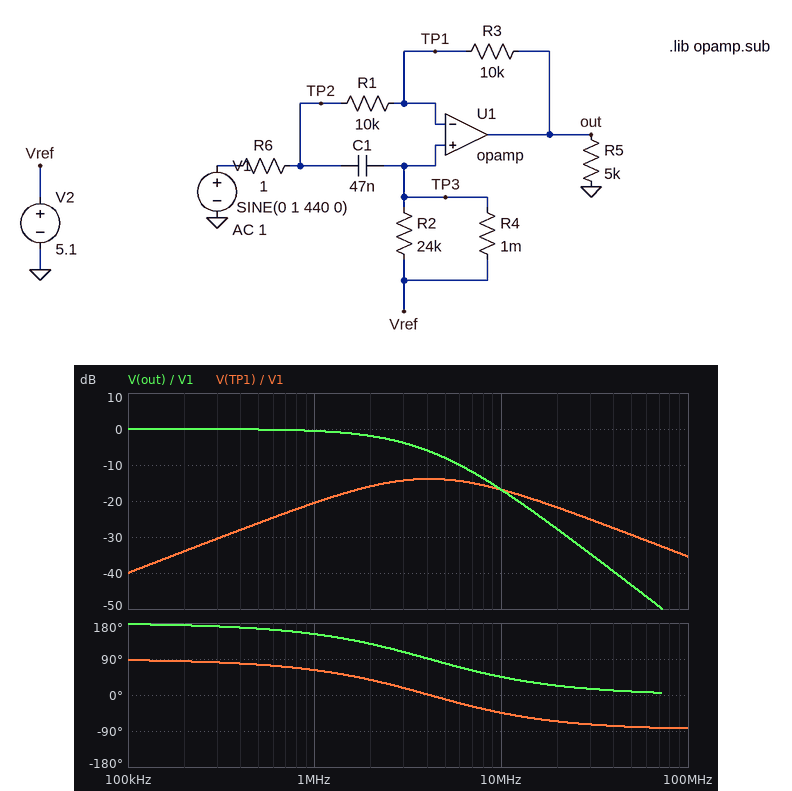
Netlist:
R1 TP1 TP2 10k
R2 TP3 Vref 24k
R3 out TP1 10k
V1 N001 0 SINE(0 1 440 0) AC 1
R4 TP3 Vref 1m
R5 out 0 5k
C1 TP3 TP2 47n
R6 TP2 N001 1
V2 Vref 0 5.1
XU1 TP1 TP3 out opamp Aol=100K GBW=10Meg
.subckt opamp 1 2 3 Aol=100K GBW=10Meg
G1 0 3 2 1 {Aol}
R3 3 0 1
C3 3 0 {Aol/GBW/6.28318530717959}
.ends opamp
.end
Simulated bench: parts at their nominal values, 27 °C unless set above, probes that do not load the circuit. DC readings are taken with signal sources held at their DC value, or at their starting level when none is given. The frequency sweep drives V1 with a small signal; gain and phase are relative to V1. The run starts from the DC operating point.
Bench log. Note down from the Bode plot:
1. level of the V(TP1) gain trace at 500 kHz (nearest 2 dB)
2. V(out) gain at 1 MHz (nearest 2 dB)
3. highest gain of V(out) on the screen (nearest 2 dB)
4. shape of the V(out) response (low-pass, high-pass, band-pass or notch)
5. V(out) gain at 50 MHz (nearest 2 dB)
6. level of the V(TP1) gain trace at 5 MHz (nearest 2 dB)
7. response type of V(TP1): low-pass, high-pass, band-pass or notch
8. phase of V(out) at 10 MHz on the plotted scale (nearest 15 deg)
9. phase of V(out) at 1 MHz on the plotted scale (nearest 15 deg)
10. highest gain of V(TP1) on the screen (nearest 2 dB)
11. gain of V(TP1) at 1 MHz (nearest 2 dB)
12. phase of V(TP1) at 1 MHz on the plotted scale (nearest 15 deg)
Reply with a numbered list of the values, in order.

1. -26 dB
2. 0 dB
3. 0 dB
4. low-pass
5. -44 dB
6. -14 dB
7. band-pass
8. 45 deg
9. 150 deg
10. -14 dB
11. -20 dB
12. 60 deg
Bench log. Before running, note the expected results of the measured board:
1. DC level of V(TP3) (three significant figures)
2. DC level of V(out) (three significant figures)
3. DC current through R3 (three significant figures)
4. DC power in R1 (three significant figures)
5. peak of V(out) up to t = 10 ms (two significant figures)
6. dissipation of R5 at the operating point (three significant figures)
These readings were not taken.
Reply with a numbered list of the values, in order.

1. 5.10 V
2. 10.2 V
3. 510 µA
4. 2.60 mW
5. 11 V
6. 20.8 mW
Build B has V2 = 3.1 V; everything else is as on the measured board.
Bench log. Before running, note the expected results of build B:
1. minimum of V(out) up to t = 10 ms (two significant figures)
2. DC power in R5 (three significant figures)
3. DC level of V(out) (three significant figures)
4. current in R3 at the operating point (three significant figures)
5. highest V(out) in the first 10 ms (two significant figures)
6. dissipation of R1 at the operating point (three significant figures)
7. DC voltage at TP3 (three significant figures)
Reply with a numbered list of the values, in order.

1. 5.2 V
2. 7.69 mW
3. 6.20 V
4. 310 µA
5. 7.2 V
6. 961 µW
7. 3.10 V
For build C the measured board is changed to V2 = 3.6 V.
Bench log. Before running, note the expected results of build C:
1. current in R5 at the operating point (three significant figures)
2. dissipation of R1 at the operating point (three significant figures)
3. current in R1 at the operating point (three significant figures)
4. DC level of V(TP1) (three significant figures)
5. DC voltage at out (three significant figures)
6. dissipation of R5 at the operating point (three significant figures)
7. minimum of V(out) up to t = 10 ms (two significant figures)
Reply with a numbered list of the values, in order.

1. 1.44 mA
2. 1.30 mW
3. 360 µA
4. 3.60 V
5. 7.20 V
6. 10.4 mW
7. 6.2 V
